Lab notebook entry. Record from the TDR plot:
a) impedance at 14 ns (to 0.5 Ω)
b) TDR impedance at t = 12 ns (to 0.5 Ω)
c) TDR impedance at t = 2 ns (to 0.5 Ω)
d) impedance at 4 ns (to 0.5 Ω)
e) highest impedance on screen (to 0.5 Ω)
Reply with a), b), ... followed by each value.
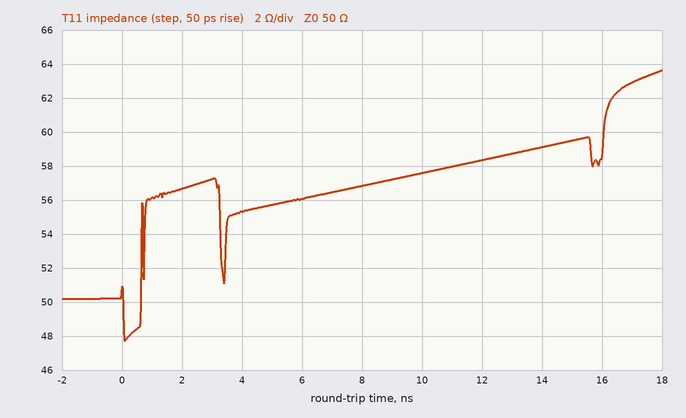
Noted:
a) 59.0 Ω
b) 58.5 Ω
c) 56.5 Ω
d) 55.5 Ω
e) 63.5 Ω
